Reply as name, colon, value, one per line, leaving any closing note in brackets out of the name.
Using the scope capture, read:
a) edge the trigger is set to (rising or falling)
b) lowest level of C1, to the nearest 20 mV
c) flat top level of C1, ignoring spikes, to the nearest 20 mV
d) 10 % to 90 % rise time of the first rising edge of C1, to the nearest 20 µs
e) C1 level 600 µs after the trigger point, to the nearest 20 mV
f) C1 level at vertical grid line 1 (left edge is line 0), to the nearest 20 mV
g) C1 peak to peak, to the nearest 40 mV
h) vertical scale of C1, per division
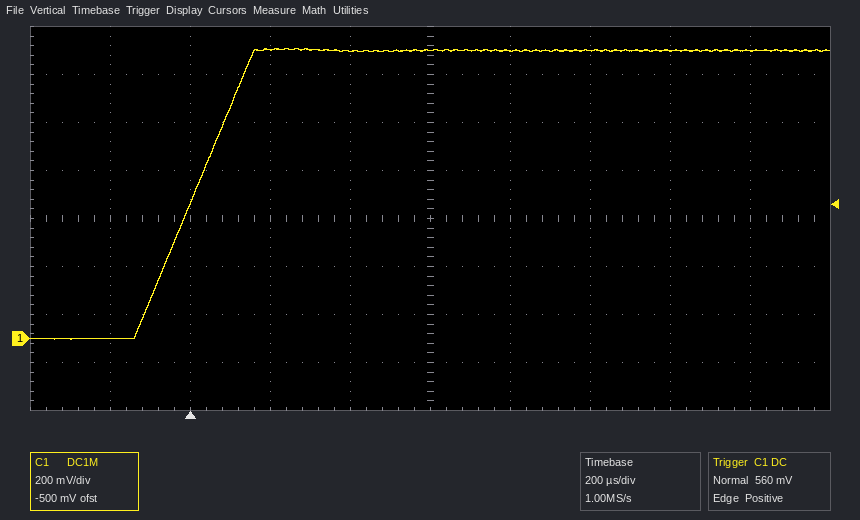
edge the trigger is set to: rising
lowest level of C1, to the nearest 20 mV: 0 mV
flat top level of C1, ignoring spikes, to the nearest 20 mV: 1.20 V
10 % to 90 % rise time of the first rising edge of C1, to the nearest 20 µs: 240 µs
C1 level 600 µs after the trigger point, to the nearest 20 mV: 1.20 V
C1 level at vertical grid line 1 (left edge is line 0), to the nearest 20 mV: 0 mV
C1 peak to peak, to the nearest 40 mV: 1.20 V
vertical scale of C1, per division: 200 mV
